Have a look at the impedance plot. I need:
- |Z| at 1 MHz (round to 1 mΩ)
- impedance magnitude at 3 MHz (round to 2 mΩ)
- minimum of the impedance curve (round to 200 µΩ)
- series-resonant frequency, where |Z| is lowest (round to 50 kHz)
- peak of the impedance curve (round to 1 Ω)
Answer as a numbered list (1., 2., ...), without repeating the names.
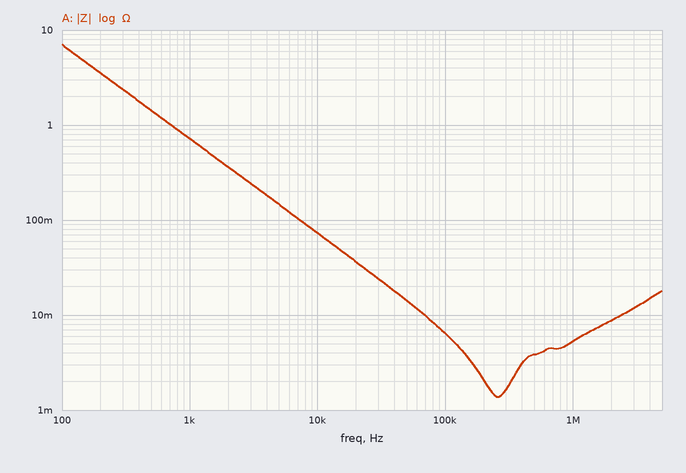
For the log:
1. 5 mΩ
2. 12 mΩ
3. 1.4 mΩ
4. 250 kHz
5. 7 Ω
